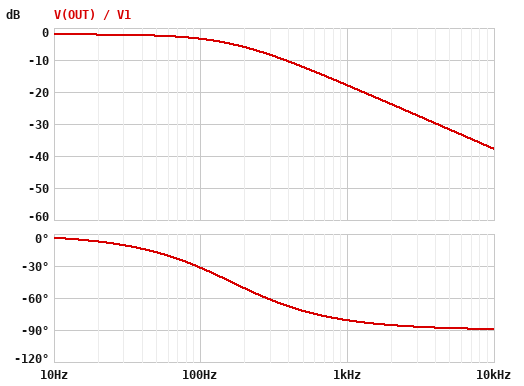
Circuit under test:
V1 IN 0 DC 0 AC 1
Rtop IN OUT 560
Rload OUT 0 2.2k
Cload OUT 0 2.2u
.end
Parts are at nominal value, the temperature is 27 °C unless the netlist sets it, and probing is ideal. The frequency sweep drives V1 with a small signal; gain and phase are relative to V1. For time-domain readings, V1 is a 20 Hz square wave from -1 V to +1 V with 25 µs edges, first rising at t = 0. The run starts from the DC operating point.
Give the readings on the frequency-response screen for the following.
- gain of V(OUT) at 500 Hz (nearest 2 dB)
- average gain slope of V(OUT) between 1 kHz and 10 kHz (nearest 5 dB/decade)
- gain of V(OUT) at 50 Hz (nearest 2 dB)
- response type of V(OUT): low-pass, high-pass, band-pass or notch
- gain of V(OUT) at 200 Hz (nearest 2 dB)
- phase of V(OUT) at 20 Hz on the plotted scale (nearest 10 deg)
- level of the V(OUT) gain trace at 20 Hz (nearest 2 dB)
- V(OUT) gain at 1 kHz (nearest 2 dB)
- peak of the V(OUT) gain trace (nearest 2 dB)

-12 dB
-20 dB/decade
-2 dB
low-pass
-6 dB
-10 deg
-2 dB
-18 dB
-2 dB
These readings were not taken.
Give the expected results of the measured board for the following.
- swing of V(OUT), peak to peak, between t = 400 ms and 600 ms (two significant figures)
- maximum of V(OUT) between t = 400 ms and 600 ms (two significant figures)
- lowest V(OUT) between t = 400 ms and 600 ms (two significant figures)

1.6 V
800 mV
-800 mV
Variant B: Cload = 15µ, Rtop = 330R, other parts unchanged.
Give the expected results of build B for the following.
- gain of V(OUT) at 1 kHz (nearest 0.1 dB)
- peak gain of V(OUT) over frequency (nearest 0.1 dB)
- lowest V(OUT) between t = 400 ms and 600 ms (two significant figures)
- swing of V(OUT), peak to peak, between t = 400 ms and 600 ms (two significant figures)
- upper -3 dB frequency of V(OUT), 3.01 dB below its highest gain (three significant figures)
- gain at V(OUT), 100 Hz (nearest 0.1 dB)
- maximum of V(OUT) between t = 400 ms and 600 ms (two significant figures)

-29.9 dB
-1.2 dB
-860 mV
1.7 V
37.0 Hz
-10.4 dB
860 mV
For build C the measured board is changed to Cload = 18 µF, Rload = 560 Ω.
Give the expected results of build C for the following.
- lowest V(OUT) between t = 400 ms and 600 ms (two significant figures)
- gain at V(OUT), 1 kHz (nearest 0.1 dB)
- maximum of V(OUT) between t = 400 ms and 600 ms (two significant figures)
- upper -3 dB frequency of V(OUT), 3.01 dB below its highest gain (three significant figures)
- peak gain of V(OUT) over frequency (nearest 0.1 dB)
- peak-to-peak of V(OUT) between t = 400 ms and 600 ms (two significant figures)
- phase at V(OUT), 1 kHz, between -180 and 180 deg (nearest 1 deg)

-490 mV
-36.0 dB
490 mV
31.6 Hz
-6.0 dB
990 mV
-88 deg
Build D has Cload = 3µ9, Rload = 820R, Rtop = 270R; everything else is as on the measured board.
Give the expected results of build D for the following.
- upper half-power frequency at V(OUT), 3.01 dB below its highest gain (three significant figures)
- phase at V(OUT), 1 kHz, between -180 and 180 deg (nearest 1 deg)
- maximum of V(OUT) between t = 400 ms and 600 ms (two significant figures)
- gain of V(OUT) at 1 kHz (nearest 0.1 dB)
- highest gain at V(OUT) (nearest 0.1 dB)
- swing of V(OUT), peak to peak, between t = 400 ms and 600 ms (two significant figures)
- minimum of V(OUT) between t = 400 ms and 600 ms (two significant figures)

201 Hz
-79 deg
750 mV
-16.6 dB
-2.5 dB
1.5 V
-750 mV
